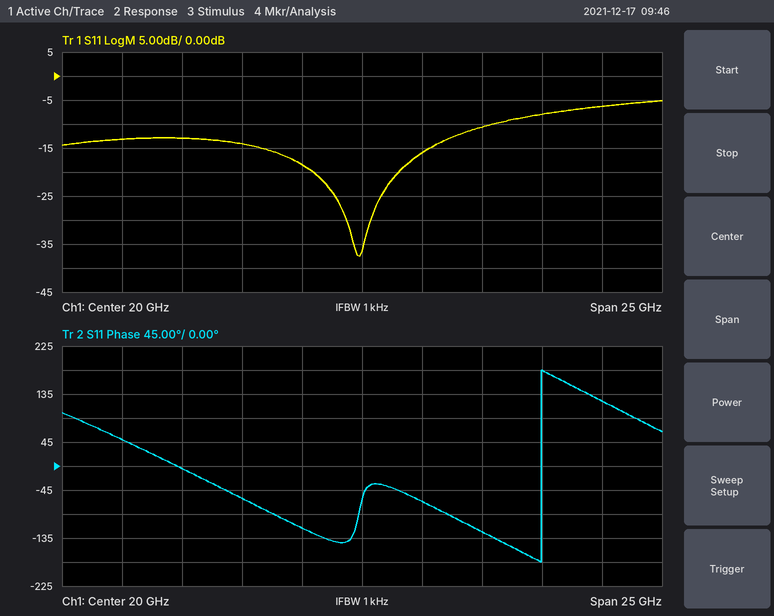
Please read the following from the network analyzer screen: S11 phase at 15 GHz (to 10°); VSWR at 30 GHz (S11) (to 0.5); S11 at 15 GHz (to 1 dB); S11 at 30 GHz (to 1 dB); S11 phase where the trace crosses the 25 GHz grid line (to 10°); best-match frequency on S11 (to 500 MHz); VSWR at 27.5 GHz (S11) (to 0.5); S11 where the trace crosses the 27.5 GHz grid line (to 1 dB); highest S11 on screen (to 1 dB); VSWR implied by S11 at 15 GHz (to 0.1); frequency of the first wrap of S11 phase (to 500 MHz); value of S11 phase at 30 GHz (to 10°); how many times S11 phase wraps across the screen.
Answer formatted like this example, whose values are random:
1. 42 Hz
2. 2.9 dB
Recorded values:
1. -60°
2. 3.0
3. -14 dB
4. -6 dB
5. -120°
6. 20.0 GHz
7. 2.5
8. -8 dB
9. -5 dB
10. 1.5
11. 27.5 GHz
12. 120°
13. 1
